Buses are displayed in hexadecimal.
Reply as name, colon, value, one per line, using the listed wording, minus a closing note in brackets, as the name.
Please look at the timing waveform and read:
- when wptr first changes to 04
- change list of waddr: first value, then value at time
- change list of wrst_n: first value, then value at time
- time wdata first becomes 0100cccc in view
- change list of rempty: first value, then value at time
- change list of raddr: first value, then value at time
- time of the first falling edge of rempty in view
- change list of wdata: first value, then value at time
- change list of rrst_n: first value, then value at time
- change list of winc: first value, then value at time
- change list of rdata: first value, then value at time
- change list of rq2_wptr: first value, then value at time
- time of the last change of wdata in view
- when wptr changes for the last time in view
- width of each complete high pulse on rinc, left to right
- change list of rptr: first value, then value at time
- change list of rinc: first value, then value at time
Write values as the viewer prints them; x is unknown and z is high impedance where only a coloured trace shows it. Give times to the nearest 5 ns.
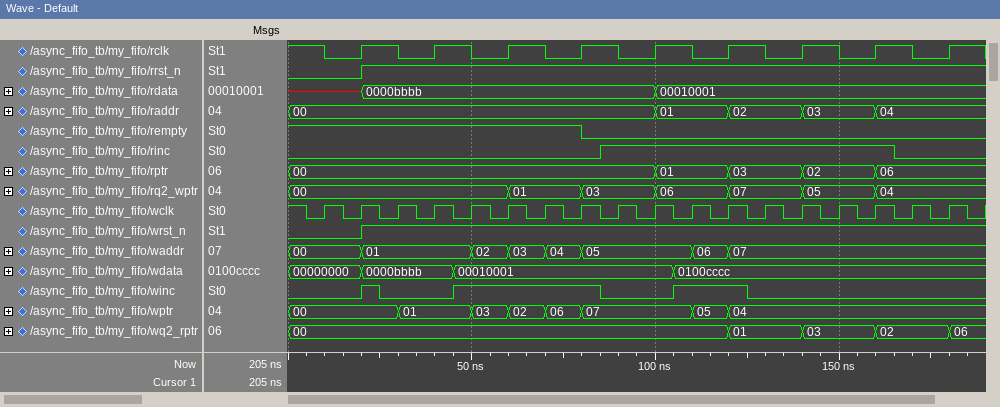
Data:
when wptr first changes to 04: 120 ns
change list of waddr: first value, then value at time: 00, 01 at 20 ns, 02 at 50 ns, 03 at 60 ns, 04 at 70 ns, 05 at 80 ns, 06 at 110 ns, 07 at 120 ns
change list of wrst_n: first value, then value at time: 0, 1 at 20 ns
time wdata first becomes 0100cccc in view: 105 ns
change list of rempty: first value, then value at time: 1, 0 at 80 ns
change list of raddr: first value, then value at time: 00, 01 at 100 ns, 02 at 120 ns, 03 at 140 ns, 04 at 160 ns
time of the first falling edge of rempty in view: 80 ns
change list of wdata: first value, then value at time: 00000000, 0000bbbb at 20 ns, 00010001 at 45 ns, 0100cccc at 105 ns
change list of rrst_n: first value, then value at time: 0, 1 at 20 ns
change list of winc: first value, then value at time: 0, 1 at 20 ns, 0 at 25 ns, 1 at 45 ns, 0 at 85 ns, 1 at 105 ns, 0 at 125 ns
change list of rdata: first value, then value at time: x, 0000bbbb at 20 ns, 00010001 at 100 ns
change list of rq2_wptr: first value, then value at time: 00, 01 at 60 ns, 03 at 80 ns, 06 at 100 ns, 07 at 120 ns, 05 at 140 ns, 04 at 160 ns
time of the last change of wdata in view: 105 ns
when wptr changes for the last time in view: 120 ns
width of each complete high pulse on rinc, left to right: 80 ns
change list of rptr: first value, then value at time: 00, 01 at 100 ns, 03 at 120 ns, 02 at 140 ns, 06 at 160 ns
change list of rinc: first value, then value at time: 0, 1 at 85 ns, 0 at 165 ns
